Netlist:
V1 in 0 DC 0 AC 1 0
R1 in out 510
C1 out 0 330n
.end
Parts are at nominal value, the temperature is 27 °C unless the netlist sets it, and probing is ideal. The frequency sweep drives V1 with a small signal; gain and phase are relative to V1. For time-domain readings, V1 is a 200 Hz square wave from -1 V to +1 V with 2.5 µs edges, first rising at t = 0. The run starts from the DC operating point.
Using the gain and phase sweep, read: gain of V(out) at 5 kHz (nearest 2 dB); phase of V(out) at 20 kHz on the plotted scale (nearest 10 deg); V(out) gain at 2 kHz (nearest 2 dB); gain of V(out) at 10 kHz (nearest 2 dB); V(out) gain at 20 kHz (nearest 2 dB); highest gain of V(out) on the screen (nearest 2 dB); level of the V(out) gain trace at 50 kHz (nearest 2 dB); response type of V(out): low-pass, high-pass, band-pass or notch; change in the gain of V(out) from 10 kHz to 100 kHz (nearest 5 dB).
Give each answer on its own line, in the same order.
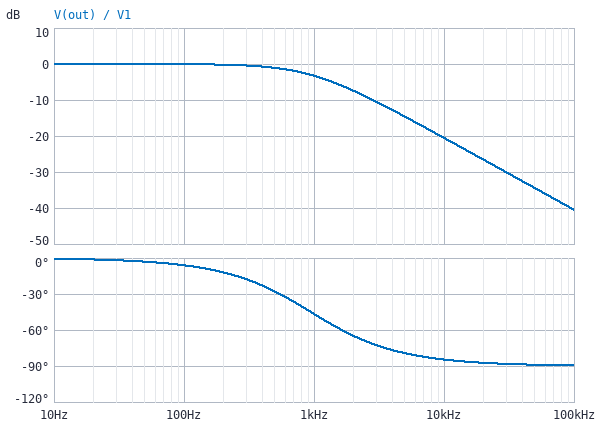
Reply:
-14 dB
-90 deg
-8 dB
-20 dB
-26 dB
0 dB
-34 dB
low-pass
-20 dB
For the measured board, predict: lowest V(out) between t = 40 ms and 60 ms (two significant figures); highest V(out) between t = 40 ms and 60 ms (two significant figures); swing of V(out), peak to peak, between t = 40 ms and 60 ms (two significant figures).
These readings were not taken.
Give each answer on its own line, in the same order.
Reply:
-1.0 V
1.0 V
2.0 V
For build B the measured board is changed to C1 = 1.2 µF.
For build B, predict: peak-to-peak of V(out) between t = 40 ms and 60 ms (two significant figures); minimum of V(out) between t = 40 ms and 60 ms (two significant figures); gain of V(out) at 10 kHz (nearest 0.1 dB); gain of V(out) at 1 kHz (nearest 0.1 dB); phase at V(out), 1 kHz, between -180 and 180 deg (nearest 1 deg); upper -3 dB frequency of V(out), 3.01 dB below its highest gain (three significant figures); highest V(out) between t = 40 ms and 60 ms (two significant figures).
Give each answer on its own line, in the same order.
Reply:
1.9 V
-970 mV
-31.7 dB
-12.0 dB
-75 deg
260 Hz
970 mV
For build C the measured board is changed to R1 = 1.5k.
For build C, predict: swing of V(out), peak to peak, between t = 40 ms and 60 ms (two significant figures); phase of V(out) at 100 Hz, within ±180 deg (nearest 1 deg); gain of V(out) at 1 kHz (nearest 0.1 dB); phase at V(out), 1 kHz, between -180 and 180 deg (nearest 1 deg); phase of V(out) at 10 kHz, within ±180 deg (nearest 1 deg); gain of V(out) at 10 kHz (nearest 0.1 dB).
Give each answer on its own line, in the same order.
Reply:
2.0 V
-17 deg
-10.3 dB
-72 deg
-88 deg
-29.9 dB
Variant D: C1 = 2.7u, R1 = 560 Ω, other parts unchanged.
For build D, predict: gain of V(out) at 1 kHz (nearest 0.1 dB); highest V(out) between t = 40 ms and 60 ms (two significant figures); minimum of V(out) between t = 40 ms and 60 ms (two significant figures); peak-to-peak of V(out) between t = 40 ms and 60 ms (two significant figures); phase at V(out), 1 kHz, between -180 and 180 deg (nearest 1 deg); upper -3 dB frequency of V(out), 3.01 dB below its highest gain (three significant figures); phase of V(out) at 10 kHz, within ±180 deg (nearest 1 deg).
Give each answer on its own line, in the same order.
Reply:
-19.6 dB
680 mV
-680 mV
1.4 V
-84 deg
105 Hz
-89 deg
